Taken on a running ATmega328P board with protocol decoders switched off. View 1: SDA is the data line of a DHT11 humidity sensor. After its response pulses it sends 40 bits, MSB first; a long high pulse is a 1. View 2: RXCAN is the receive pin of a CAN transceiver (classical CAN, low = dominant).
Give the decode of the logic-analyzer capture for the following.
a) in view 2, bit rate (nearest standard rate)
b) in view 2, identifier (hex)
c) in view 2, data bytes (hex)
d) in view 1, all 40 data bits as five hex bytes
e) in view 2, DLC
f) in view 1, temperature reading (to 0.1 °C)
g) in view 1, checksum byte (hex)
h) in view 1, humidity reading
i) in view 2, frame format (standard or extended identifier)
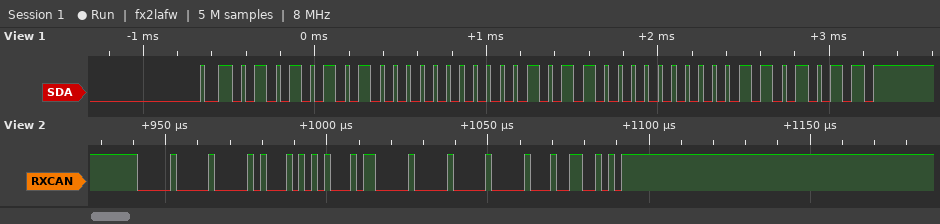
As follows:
500 kbit/s
0x000
55 16 00 00
55 00 16 00 6B
4
22.0 °C
0x6B
85 %
standard
